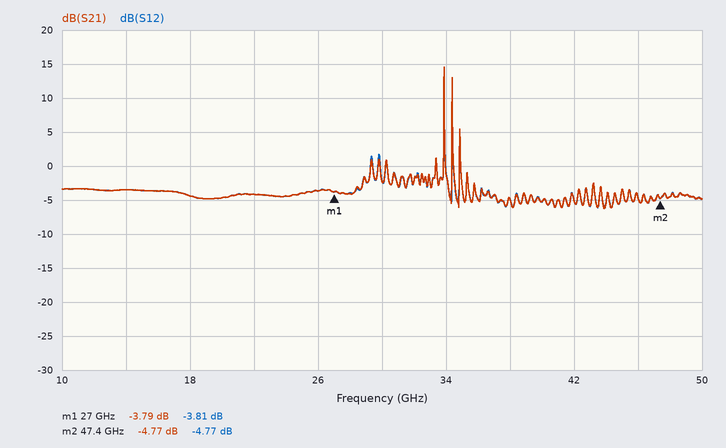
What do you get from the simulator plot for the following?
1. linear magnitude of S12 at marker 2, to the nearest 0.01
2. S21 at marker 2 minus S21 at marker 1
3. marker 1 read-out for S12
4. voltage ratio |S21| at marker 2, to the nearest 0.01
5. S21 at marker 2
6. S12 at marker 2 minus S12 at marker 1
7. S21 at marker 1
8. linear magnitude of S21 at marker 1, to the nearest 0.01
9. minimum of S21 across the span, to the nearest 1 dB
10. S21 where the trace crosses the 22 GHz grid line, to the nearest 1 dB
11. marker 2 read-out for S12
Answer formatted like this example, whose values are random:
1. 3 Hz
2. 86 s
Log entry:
1. 0.58
2. -0.98 dB
3. -3.81 dB
4. 0.58
5. -4.77 dB
6. -0.96 dB
7. -3.79 dB
8. 0.65
9. -6 dB
10. -4 dB
11. -4.77 dB
